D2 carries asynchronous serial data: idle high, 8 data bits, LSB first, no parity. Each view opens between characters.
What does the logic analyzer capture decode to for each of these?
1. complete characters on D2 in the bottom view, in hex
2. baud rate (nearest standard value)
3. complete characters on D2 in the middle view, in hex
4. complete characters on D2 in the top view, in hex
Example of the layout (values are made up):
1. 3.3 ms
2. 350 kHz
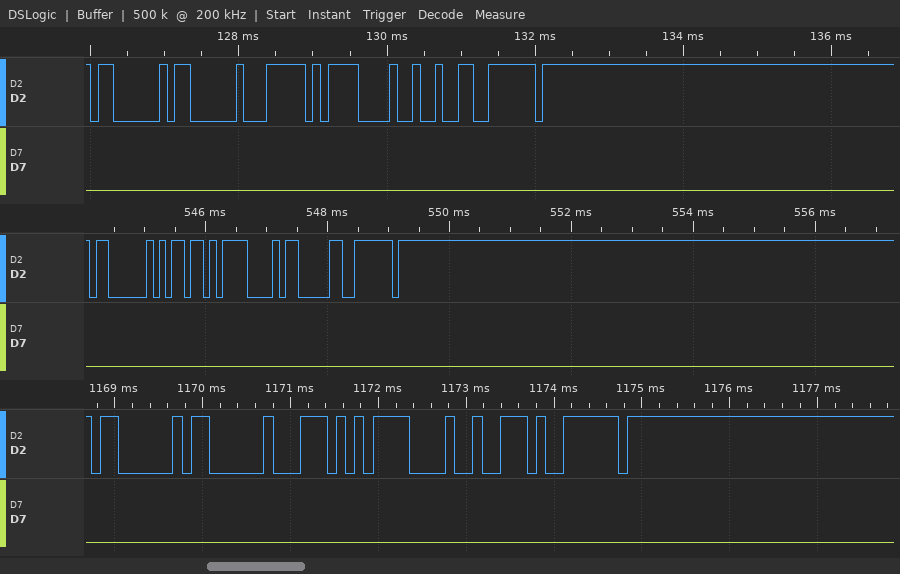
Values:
1. 03, 03, 5C, 0F, 72, 7E
2. 9600 baud
3. 03, 6D, 0F, 83, 7E
4. 03, 03, 7C, 0F, 92, 7E
